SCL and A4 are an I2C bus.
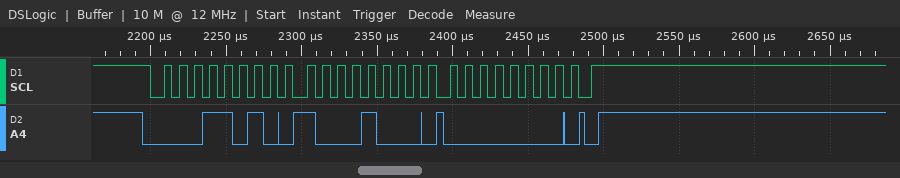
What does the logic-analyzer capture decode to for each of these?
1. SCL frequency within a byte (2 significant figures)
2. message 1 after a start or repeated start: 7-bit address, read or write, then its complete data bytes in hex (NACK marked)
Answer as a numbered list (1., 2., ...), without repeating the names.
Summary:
1. 100 kHz
2. 0x0D write: 88 00
